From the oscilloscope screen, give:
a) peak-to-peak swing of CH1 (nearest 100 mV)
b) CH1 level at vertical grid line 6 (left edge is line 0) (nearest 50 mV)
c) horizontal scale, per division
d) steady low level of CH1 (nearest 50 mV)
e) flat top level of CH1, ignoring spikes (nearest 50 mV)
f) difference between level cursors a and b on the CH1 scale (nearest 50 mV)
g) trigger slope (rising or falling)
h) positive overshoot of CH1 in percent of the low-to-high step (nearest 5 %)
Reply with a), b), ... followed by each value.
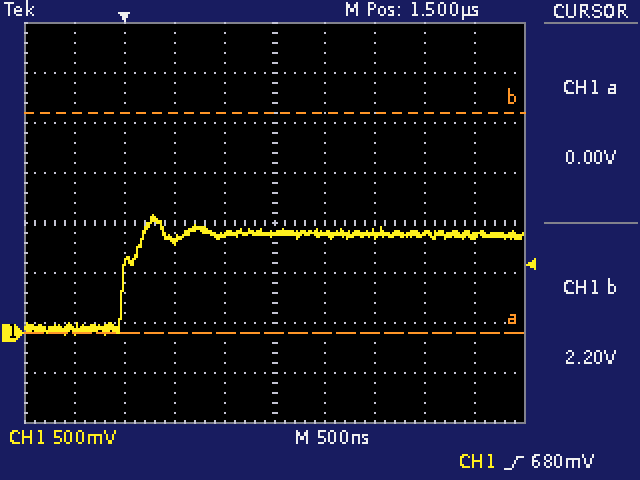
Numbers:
a) 1.20 V
b) 1.00 V
c) 500 ns
d) 50 mV
e) 1.00 V
f) 2.20 V
g) rising
h) 20 %
